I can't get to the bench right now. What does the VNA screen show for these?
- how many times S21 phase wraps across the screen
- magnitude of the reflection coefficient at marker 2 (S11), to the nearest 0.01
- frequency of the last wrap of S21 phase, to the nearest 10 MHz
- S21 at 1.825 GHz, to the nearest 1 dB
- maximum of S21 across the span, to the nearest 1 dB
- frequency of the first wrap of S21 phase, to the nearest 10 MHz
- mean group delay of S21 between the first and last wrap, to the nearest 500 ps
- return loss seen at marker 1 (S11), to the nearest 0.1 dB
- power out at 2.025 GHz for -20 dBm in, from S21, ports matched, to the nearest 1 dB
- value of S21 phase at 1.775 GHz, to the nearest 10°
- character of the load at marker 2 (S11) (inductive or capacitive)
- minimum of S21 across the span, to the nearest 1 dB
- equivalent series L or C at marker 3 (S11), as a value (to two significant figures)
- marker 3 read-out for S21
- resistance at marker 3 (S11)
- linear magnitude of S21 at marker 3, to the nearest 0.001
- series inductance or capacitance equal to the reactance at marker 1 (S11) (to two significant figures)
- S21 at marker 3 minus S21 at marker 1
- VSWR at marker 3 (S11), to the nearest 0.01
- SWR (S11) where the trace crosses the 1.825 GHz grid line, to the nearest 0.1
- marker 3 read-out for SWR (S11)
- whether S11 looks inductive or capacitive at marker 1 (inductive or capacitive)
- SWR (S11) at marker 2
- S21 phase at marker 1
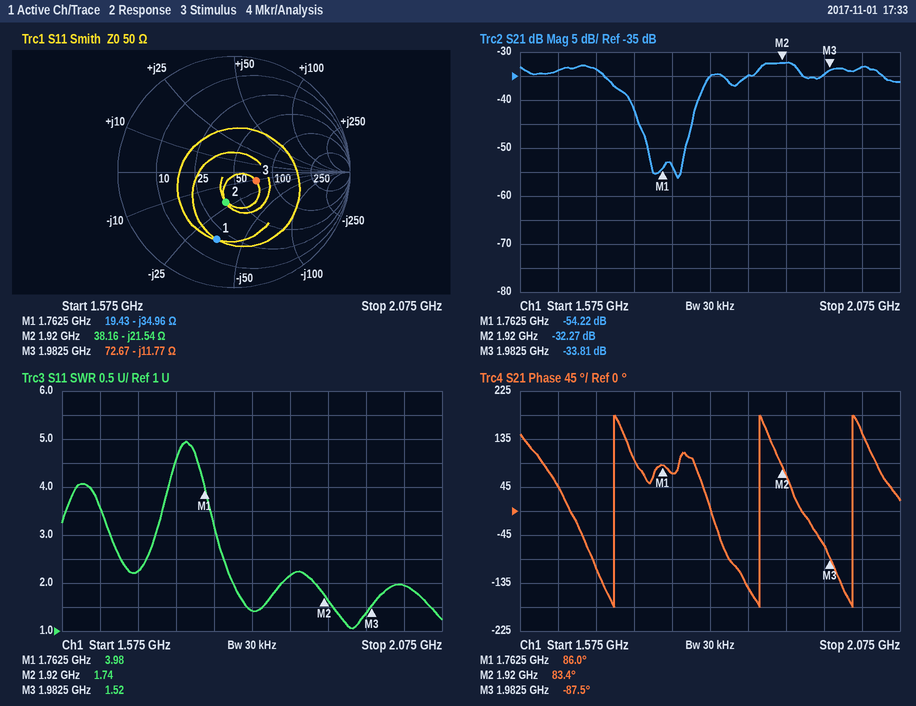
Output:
3
0.27
2.01 GHz
-35 dB
-32 dB
1.70 GHz
6.5 ns
4.5 dB
-53 dBm
70°
capacitive
-56 dB
6.8 pF
-33.81 dB
72.67 Ω
0.020
2.6 pF
20.41 dB
1.52
1.4
1.52
capacitive
1.74
86.0°
